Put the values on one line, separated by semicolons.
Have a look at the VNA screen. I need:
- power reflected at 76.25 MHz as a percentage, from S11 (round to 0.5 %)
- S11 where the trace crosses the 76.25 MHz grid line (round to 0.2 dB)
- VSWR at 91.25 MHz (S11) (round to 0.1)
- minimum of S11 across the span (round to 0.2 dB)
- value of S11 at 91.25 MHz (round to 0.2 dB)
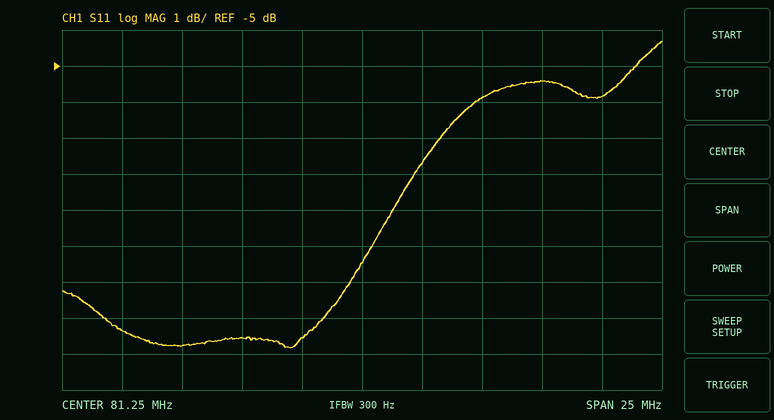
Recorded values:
5.5 %; -12.6 dB; 3.1; -12.8 dB; -5.8 dB
